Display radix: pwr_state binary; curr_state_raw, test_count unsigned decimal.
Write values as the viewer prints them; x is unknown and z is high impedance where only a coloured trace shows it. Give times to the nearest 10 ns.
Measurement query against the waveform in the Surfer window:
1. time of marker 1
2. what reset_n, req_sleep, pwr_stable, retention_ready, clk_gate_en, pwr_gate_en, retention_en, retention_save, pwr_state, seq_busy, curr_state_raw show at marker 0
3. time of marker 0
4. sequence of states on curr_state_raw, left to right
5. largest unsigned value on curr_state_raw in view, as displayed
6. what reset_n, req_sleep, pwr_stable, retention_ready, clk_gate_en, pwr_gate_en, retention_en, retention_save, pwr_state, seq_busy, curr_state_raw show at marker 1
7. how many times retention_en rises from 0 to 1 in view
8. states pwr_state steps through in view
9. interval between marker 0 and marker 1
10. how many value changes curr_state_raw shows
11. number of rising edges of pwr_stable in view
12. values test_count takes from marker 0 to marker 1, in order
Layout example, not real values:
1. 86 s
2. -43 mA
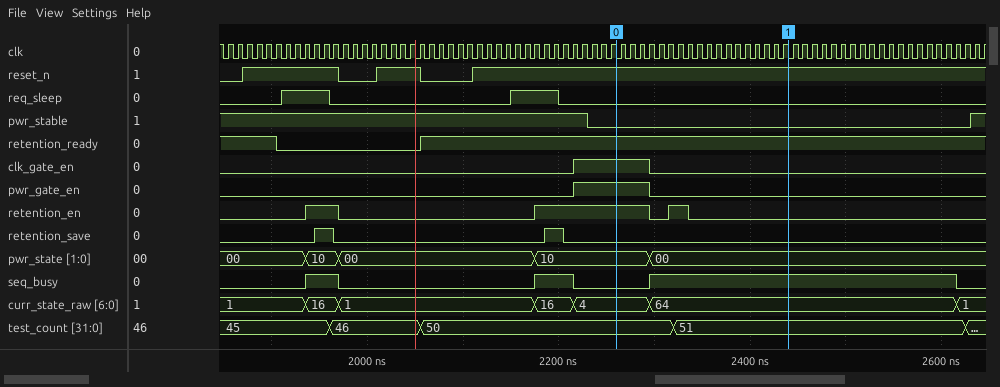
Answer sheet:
1. 2440 ns
2. reset_n=1, req_sleep=0, pwr_stable=0, retention_ready=1, clk_gate_en=1, pwr_gate_en=1, retention_en=1, retention_save=0, pwr_state=10, seq_busy=0, curr_state_raw=4
3. 2260 ns
4. 1, 16, 1, 16, 4, 64, 1
5. 64
6. reset_n=1, req_sleep=0, pwr_stable=0, retention_ready=1, clk_gate_en=0, pwr_gate_en=0, retention_en=0, retention_save=0, pwr_state=00, seq_busy=1, curr_state_raw=64
7. 3
8. 00, 10, 00, 10, 00
9. 180 ns
10. 6
11. 1
12. 50, 51
